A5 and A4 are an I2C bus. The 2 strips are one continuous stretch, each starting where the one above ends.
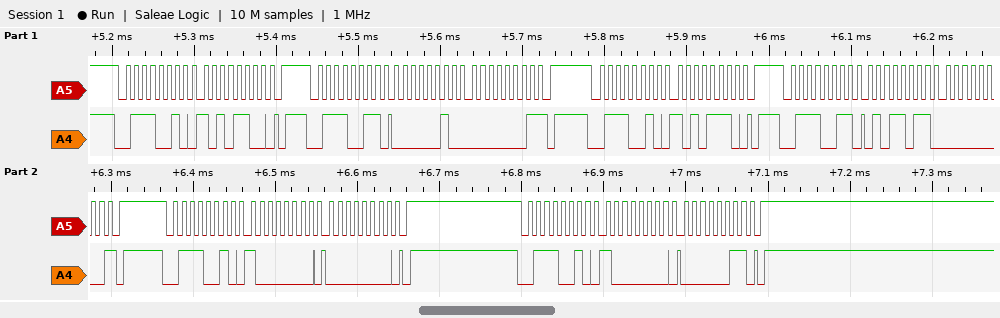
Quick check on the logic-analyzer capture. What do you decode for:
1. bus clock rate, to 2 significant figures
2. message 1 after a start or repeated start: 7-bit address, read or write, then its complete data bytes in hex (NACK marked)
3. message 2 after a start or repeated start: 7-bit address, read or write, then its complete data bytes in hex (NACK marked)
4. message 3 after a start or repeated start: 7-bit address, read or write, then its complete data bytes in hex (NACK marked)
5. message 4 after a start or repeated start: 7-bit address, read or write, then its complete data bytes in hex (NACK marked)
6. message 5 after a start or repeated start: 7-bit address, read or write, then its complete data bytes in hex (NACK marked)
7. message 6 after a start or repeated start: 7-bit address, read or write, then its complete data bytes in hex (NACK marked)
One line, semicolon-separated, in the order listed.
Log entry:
100 kHz; 0x39 write: AC; 0x39 read: 02 01 NACK; 0x39 write: AE; 0x39 read: 5B 00 NACK; 0x39 write: 80 00; 0x39 write: 80 03
